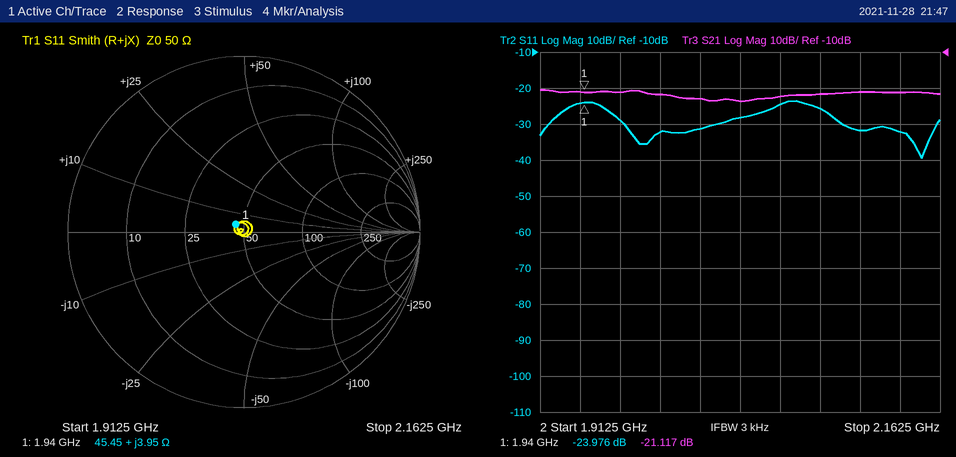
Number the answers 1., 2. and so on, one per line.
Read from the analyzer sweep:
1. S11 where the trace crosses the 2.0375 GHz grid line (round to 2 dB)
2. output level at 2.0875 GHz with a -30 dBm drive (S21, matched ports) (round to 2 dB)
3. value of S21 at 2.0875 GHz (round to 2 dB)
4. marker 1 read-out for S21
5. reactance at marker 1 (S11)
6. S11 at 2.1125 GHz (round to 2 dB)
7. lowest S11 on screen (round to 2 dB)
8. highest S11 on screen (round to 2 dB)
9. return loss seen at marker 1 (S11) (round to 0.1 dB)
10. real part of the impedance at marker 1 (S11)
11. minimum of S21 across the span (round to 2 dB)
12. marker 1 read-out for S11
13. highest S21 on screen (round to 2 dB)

1. -28 dB
2. -52 dBm
3. -22 dB
4. -21.117 dB
5. +3.95 Ω
6. -32 dB
7. -40 dB
8. -24 dB
9. 24.0 dB
10. 45.45 Ω
11. -24 dB
12. -23.976 dB
13. -20 dB
